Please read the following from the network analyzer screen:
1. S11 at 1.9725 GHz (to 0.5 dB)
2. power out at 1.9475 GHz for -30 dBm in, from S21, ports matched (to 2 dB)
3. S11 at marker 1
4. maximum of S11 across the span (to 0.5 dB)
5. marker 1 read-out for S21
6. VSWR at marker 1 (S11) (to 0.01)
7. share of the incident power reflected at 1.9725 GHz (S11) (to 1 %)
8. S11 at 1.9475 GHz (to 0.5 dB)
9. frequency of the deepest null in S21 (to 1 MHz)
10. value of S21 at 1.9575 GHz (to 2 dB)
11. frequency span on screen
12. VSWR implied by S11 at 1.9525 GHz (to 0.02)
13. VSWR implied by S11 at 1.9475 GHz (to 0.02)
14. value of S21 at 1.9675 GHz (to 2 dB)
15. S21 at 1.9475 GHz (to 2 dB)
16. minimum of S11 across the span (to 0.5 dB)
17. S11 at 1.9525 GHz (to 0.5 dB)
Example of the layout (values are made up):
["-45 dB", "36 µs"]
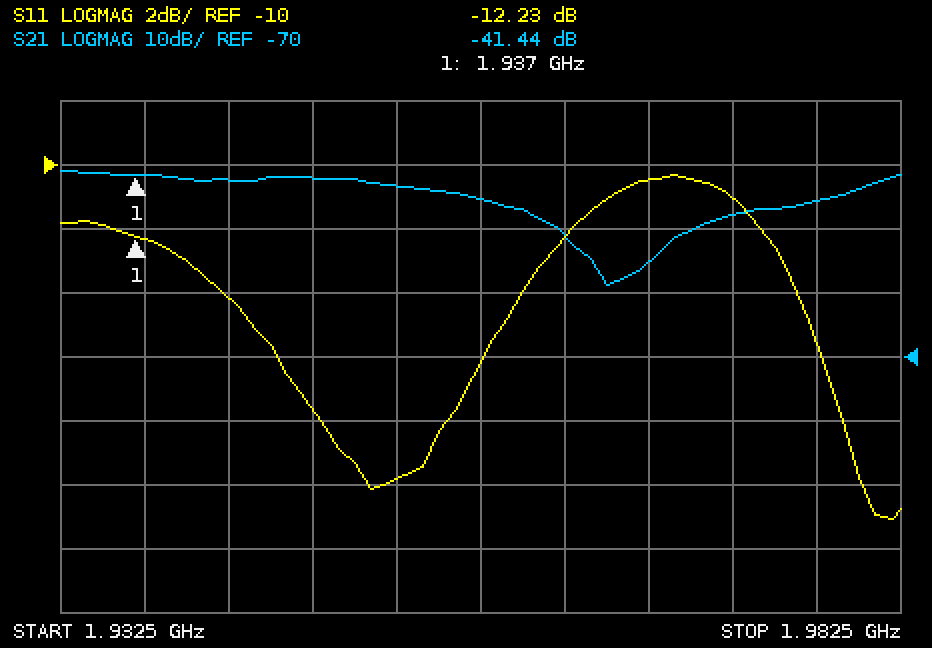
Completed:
["-11.0 dB", "-72 dBm", "-12.23 dB", "-10.5 dB", "-41.44 dB", "1.65", "8 %", "-17.5 dB", "1.965 GHz", "-46 dB", "50 MHz", "1.22", "1.30", "-56 dB", "-42 dB", "-21.0 dB", "-20.0 dB"]
